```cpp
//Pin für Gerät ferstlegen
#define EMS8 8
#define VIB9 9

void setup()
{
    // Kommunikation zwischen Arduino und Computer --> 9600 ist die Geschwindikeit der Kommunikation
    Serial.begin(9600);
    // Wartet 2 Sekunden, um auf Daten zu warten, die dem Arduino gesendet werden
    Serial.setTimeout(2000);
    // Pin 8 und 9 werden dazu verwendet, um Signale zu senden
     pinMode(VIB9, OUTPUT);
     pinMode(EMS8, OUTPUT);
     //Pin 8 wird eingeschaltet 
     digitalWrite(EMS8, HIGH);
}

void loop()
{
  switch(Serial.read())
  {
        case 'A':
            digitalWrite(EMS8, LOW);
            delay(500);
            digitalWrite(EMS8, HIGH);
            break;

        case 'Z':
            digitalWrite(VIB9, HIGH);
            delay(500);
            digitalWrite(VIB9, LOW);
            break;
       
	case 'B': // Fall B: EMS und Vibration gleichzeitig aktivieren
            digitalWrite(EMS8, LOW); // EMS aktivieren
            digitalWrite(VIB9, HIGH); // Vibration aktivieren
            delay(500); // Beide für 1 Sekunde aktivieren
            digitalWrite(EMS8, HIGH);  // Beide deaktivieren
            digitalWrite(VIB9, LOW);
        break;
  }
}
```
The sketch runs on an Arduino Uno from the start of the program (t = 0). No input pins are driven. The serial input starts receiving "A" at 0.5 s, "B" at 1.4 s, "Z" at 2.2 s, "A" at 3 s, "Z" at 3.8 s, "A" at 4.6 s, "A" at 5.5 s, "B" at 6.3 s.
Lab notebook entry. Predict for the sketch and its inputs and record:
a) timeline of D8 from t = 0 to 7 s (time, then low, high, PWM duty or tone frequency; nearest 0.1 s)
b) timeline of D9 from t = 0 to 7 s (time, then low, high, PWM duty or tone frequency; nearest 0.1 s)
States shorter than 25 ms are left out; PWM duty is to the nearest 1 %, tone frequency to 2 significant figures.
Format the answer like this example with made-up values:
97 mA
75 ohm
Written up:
0 s high; 0.5 s low; 1 s high; 1.4 s low; 1.9 s high; 3 s low; 3.5 s high; 4.6 s low; 5.1 s high; 5.5 s low; 6 s high; 6.3 s low; 6.8 s high
0 s low; 1.4 s high; 1.9 s low; 2.2 s high; 2.7 s low; 3.8 s high; 4.3 s low; 6.3 s high; 6.8 s low
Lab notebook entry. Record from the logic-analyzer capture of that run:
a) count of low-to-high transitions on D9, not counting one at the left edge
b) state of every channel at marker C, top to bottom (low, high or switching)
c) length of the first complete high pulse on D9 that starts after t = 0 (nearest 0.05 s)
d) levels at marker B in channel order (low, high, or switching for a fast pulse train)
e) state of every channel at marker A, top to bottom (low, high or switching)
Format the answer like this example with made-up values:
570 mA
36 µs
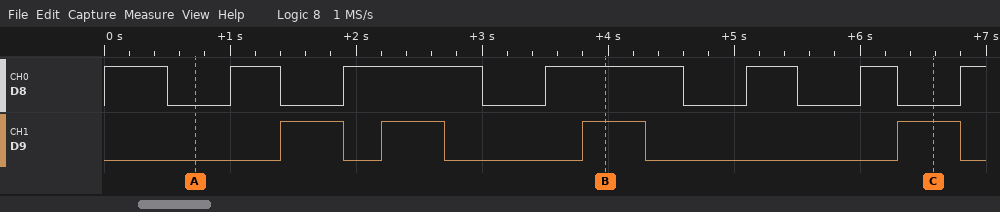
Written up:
4
D8 low, D9 high
0.50 s
D8 high, D9 high
D8 low, D9 low
